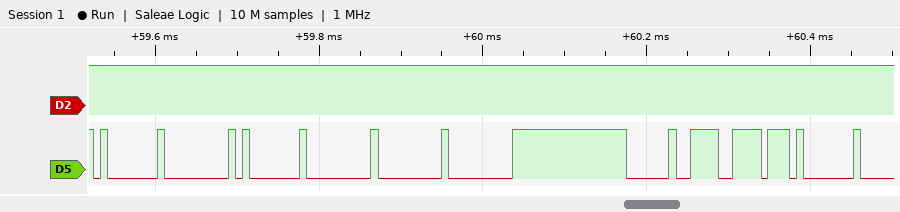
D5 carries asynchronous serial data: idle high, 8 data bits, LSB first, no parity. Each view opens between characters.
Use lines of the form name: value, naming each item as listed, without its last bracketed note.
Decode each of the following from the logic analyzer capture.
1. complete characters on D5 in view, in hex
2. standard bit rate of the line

complete characters on D5 in view, in hex: 01, 00, 01, 00, 00, 00, 20, DE, 01
standard bit rate of the line: 115200 baud
